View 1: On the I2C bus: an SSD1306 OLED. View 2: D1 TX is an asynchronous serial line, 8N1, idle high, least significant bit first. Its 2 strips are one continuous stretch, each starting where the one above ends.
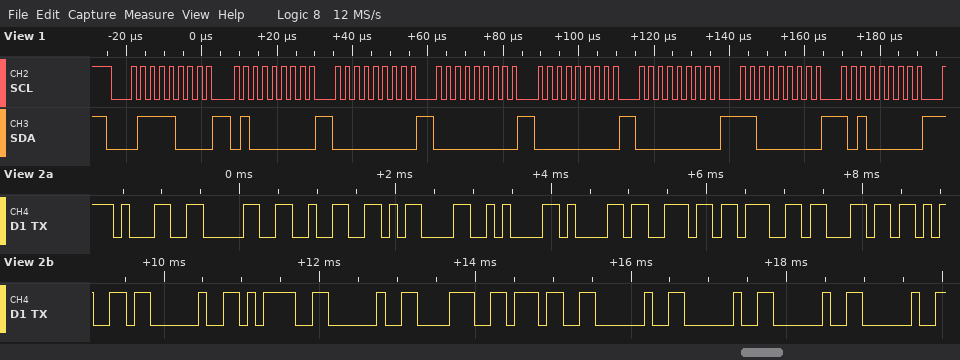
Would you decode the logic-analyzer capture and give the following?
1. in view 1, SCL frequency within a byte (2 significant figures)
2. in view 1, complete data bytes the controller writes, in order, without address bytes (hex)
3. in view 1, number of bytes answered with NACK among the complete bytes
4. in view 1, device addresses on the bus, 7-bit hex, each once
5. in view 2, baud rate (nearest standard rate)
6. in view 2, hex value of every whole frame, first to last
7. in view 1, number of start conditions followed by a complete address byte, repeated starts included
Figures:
400 kHz
40 00 00 00 00 C0 A0
0
0x3C
9600 baud
31 30 32 0D 0A 61 6E 67 6C 65 20 3D 20 38 37 20 20 20 20
1
